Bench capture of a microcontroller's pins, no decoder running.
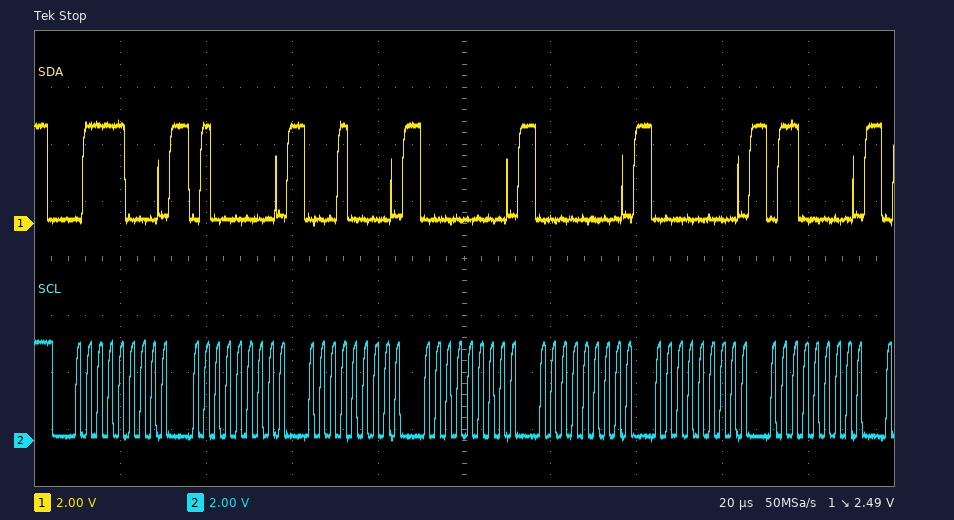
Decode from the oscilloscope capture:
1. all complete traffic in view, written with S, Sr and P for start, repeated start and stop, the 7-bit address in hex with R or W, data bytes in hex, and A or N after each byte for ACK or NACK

S 3CW A 40 A 10 A 00 A 00 A 00 A 60 A
